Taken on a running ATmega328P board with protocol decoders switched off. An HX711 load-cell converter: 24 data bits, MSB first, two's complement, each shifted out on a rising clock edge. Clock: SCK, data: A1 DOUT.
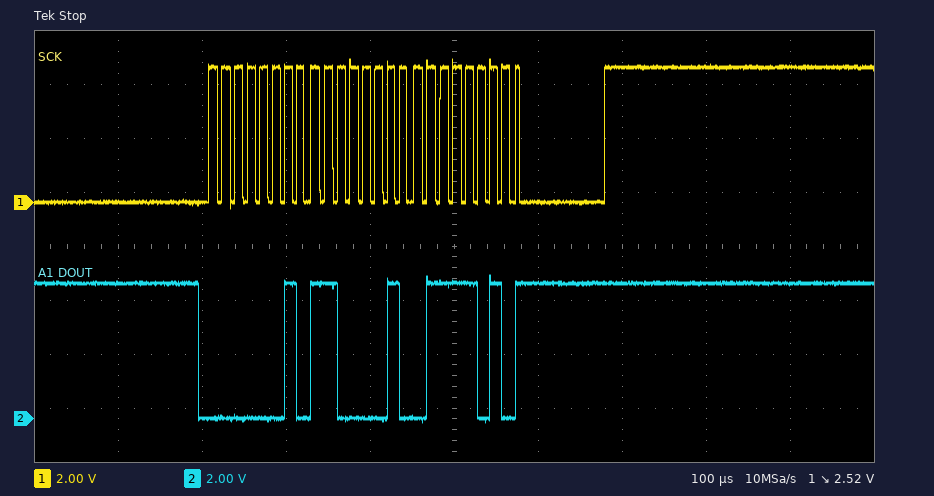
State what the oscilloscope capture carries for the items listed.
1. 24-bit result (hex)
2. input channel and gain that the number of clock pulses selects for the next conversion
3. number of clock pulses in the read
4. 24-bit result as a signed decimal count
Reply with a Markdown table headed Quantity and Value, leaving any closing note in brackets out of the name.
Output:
| Quantity | Value |
|---|---|
| 24-bit result | 0x02C27A |
| input channel and gain that the number of clock pulses selects for the next conversion | channel B, gain 32 |
| number of clock pulses in the read | 26 |
| 24-bit result as a signed decimal count | 180858 |
